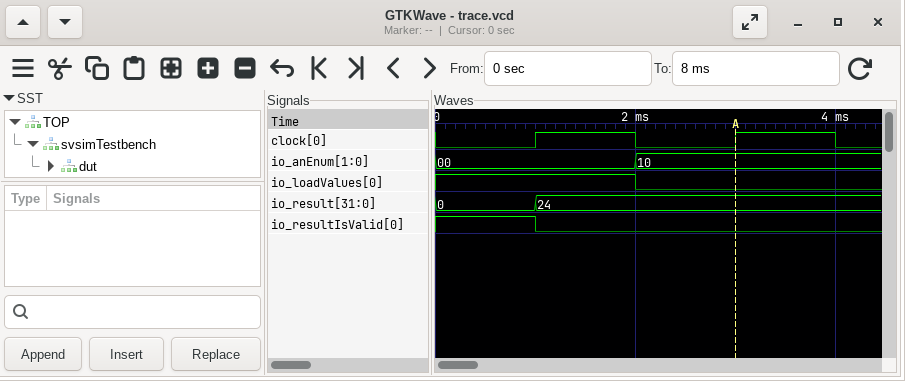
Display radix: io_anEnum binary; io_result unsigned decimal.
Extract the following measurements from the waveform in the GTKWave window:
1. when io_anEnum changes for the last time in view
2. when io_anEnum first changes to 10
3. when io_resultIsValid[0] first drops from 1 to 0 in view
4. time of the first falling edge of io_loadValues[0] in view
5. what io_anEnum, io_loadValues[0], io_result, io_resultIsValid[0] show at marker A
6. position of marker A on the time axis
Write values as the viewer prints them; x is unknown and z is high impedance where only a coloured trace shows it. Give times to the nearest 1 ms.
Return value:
2 ms
2 ms
1 ms
2 ms
io_anEnum=10, io_loadValues[0]=0, io_result=24, io_resultIsValid[0]=0
3 ms
